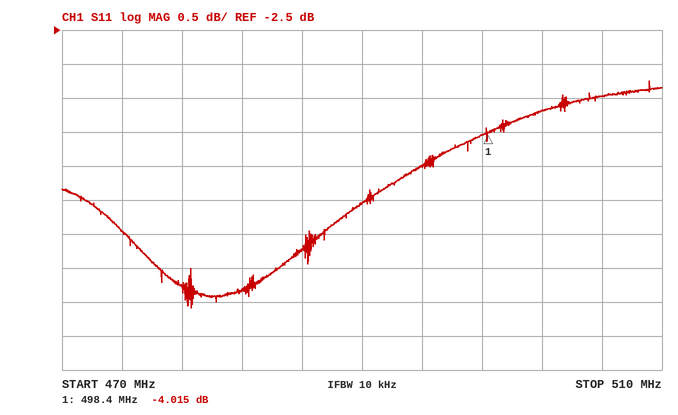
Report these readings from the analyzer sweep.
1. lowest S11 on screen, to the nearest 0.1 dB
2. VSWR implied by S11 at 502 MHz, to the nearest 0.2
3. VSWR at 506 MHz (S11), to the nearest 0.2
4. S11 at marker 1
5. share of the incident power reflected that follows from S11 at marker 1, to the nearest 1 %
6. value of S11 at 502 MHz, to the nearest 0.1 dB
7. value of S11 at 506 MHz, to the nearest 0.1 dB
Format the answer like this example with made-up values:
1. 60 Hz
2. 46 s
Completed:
1. -6.6 dB
2. 4.8
3. 5.0
4. -4.015 dB
5. 40 %
6. -3.7 dB
7. -3.5 dB
